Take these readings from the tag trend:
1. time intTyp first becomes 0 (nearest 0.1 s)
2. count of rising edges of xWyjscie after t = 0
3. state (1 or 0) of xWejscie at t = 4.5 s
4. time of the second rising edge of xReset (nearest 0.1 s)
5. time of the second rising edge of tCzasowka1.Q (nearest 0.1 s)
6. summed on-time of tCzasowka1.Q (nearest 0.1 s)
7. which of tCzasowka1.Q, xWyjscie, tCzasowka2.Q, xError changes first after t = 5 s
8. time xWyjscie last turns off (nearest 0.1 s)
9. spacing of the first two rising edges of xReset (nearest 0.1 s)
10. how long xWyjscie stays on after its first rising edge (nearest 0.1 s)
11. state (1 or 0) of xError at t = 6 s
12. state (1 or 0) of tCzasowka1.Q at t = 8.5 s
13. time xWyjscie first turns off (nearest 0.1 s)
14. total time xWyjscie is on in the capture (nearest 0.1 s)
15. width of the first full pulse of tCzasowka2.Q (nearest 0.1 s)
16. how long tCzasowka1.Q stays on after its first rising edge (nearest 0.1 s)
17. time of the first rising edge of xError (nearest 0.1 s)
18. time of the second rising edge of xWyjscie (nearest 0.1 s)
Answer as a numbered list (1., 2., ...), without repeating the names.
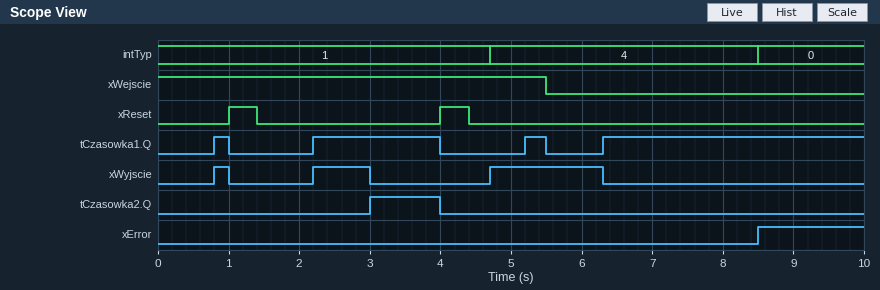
1. 8.5 s
2. 3
3. 1
4. 4.0 s
5. 2.2 s
6. 6.0 s
7. tCzasowka1.Q
8. 6.3 s
9. 3.0 s
10. 0.2 s
11. 0
12. 1
13. 1.0 s
14. 2.6 s
15. 1.0 s
16. 0.2 s
17. 8.5 s
18. 2.2 s
